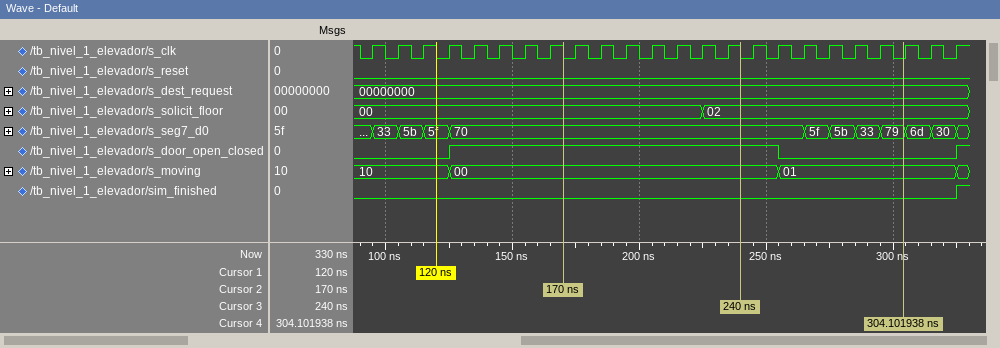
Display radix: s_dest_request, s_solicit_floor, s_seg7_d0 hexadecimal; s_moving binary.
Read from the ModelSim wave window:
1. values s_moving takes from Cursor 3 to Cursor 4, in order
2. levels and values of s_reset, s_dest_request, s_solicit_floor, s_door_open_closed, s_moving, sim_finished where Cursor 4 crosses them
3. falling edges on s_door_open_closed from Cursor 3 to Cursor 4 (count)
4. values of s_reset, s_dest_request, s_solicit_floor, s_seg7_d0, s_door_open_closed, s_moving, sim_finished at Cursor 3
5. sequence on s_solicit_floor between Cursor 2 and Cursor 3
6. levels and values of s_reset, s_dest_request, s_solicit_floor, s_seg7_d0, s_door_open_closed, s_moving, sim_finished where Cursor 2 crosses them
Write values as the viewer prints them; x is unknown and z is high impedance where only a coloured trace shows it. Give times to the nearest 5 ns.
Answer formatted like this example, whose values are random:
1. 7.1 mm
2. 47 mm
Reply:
1. 00, 01
2. s_reset=0, s_dest_request=00000000, s_solicit_floor=02, s_door_open_closed=0, s_moving=01, sim_finished=0
3. 1
4. s_reset=0, s_dest_request=00000000, s_solicit_floor=02, s_seg7_d0=70, s_door_open_closed=1, s_moving=00, sim_finished=0
5. 00, 02
6. s_reset=0, s_dest_request=00000000, s_solicit_floor=00, s_seg7_d0=70, s_door_open_closed=1, s_moving=00, sim_finished=0
